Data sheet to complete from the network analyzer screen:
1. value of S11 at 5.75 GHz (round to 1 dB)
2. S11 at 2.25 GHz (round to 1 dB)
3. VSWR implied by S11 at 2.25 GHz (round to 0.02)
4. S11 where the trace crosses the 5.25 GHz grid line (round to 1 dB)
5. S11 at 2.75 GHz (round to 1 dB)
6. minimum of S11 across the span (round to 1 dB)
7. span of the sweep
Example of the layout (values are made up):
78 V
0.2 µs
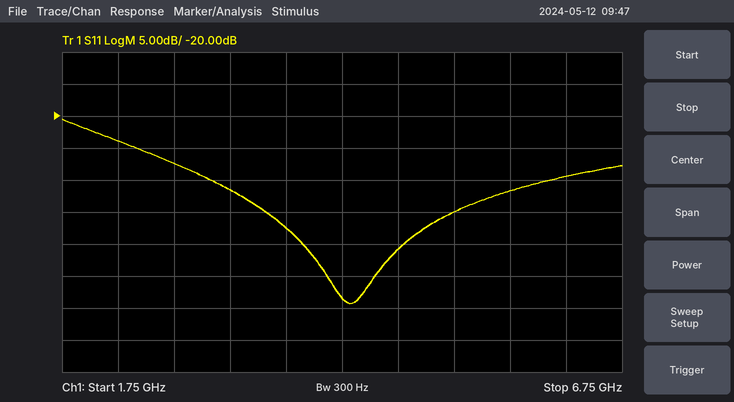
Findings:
-32 dB
-24 dB
1.14
-35 dB
-27 dB
-49 dB
5 GHz
